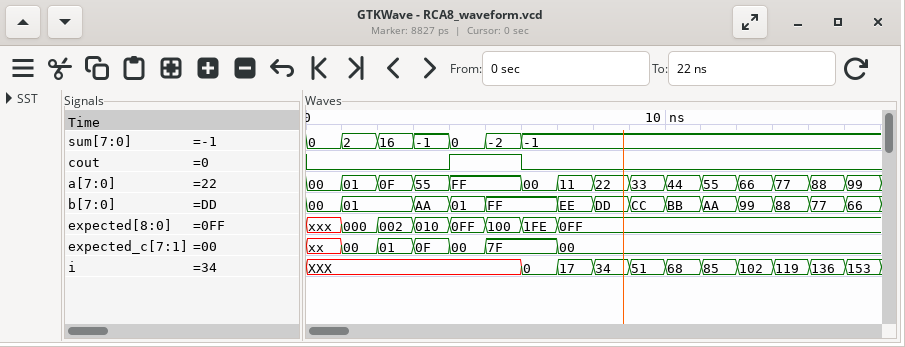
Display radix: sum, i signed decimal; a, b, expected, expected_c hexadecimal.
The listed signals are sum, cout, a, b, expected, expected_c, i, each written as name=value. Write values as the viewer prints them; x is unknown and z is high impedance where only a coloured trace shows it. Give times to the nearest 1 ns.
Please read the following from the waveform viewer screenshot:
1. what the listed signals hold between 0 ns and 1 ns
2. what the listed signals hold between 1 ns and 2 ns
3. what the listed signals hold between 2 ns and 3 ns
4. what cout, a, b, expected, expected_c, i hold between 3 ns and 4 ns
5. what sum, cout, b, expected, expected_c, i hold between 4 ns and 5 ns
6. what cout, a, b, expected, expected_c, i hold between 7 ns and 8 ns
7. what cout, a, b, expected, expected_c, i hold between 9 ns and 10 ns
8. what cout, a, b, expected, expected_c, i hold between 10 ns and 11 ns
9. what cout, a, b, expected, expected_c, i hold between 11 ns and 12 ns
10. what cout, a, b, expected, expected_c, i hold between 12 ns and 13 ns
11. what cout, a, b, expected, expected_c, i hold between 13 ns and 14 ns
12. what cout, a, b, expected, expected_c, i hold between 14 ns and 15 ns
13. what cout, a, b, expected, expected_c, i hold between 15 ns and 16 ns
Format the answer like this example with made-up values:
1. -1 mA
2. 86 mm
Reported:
1. sum=0, cout=0, a=00, b=00, expected=xxx, expected_c=xx, i=XXX
2. sum=2, cout=0, a=01, b=01, expected=000, expected_c=00, i=XXX
3. sum=16, cout=0, a=0F, b=01, expected=002, expected_c=01, i=XXX
4. cout=0, a=55, b=AA, expected=010, expected_c=0F, i=XXX
5. sum=0, cout=1, b=01, expected=0FF, expected_c=00, i=XXX
6. cout=0, a=11, b=EE, expected=0FF, expected_c=00, i=17
7. cout=0, a=33, b=CC, expected=0FF, expected_c=00, i=51
8. cout=0, a=44, b=BB, expected=0FF, expected_c=00, i=68
9. cout=0, a=55, b=AA, expected=0FF, expected_c=00, i=85
10. cout=0, a=66, b=99, expected=0FF, expected_c=00, i=102
11. cout=0, a=77, b=88, expected=0FF, expected_c=00, i=119
12. cout=0, a=88, b=77, expected=0FF, expected_c=00, i=136
13. cout=0, a=99, b=66, expected=0FF, expected_c=00, i=153
